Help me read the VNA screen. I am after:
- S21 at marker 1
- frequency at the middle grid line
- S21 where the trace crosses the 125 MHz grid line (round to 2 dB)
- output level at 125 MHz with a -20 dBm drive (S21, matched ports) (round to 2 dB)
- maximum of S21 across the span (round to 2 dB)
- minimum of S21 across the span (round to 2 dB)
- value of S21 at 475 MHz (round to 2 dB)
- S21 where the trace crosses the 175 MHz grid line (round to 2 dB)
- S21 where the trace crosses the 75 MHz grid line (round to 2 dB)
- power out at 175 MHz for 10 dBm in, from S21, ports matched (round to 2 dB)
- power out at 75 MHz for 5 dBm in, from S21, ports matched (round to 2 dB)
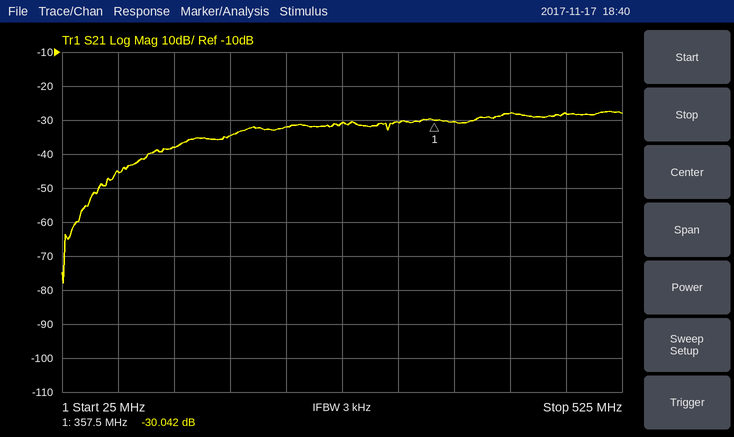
-30.042 dB
275 MHz
-38 dB
-58 dBm
-28 dB
-78 dB
-28 dB
-34 dB
-46 dB
-24 dBm
-40 dBm
